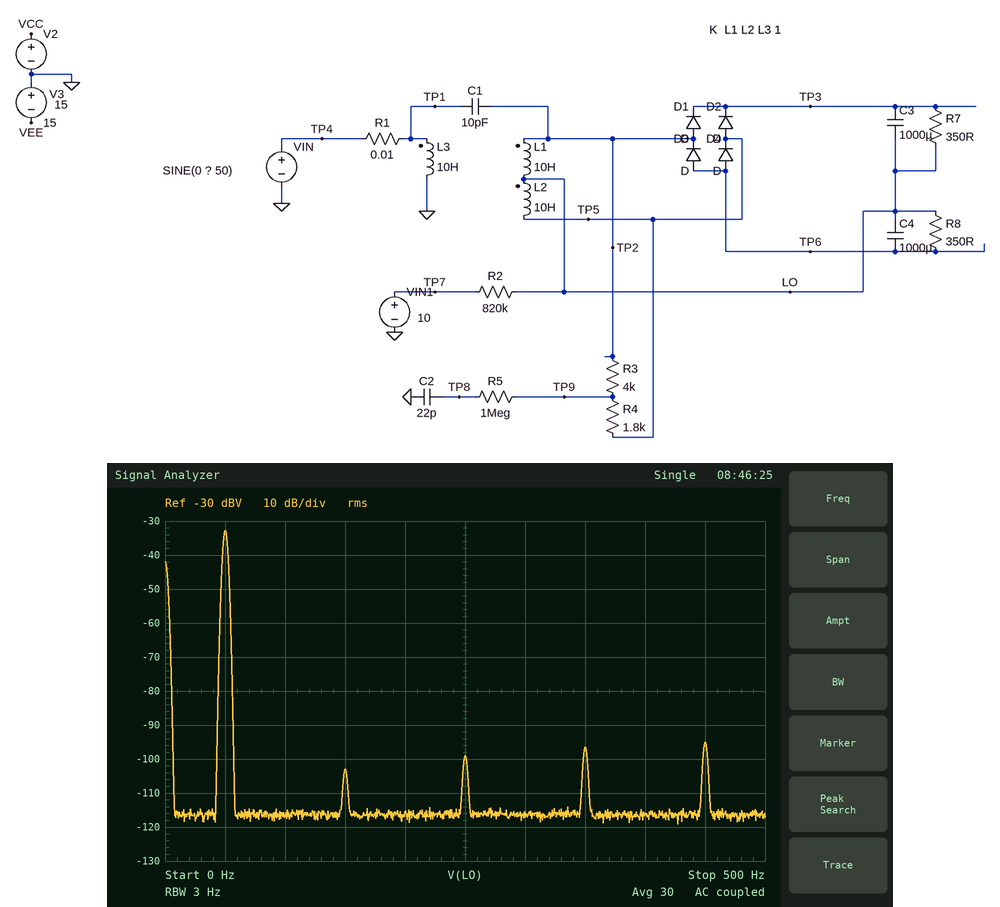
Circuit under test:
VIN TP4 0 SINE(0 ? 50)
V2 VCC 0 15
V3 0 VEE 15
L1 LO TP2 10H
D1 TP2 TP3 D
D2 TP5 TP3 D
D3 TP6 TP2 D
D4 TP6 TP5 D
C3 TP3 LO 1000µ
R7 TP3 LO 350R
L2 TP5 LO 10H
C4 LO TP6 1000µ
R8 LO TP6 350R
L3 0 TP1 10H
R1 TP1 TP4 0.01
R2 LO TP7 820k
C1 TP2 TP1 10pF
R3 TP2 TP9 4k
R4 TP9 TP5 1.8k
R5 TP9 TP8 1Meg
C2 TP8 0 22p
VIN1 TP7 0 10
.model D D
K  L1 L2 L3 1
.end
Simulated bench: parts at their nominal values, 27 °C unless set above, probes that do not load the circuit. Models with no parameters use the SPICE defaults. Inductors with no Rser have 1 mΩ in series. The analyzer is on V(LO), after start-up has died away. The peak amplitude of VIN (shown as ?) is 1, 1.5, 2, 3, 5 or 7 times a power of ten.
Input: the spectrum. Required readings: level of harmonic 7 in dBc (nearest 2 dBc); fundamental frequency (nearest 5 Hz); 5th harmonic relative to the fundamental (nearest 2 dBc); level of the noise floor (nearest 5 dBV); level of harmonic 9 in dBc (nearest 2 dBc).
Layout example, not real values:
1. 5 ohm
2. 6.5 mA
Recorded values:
1. -64 dBc
2. 50 Hz
3. -66 dBc
4. -115 dBV
5. -62 dBc
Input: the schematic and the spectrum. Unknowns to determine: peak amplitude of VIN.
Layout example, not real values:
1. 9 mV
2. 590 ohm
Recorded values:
1. 15 V
